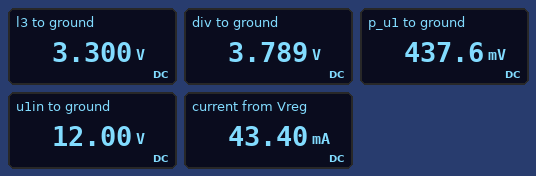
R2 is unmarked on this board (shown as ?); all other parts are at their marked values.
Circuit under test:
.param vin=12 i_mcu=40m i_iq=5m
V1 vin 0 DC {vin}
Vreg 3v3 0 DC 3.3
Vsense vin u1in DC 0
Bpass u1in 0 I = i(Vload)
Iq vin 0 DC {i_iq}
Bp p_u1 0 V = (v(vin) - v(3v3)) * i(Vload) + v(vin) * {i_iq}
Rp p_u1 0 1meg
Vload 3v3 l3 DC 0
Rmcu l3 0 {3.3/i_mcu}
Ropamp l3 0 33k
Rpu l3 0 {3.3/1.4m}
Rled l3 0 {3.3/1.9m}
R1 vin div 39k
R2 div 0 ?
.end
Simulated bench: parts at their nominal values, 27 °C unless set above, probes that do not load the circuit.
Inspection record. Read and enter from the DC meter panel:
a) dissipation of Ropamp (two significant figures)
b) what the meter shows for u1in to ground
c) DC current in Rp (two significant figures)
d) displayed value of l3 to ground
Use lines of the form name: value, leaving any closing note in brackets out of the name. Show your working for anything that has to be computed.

dissipation of Ropamp: (3.3 V)^2 / 33 kΩ = 330 µW
what the meter shows for u1in to ground: 12.00 V
DC current in Rp: (437.6 mV) / 1 MΩ = 440 nA
displayed value of l3 to ground: 3.300 V
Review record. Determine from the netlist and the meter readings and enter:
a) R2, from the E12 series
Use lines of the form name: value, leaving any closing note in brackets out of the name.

R2, from the E12 series: 18 kΩ
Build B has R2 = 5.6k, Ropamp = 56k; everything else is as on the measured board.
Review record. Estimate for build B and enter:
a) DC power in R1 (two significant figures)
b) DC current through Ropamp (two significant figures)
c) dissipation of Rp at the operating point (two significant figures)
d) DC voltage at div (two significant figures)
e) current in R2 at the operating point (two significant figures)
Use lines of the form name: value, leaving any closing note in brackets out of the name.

DC power in R1: 2.8 mW
DC current through Ropamp: 59 µA
dissipation of Rp at the operating point: 190 nW
DC voltage at div: 1.5 V
current in R2 at the operating point: 270 µA
